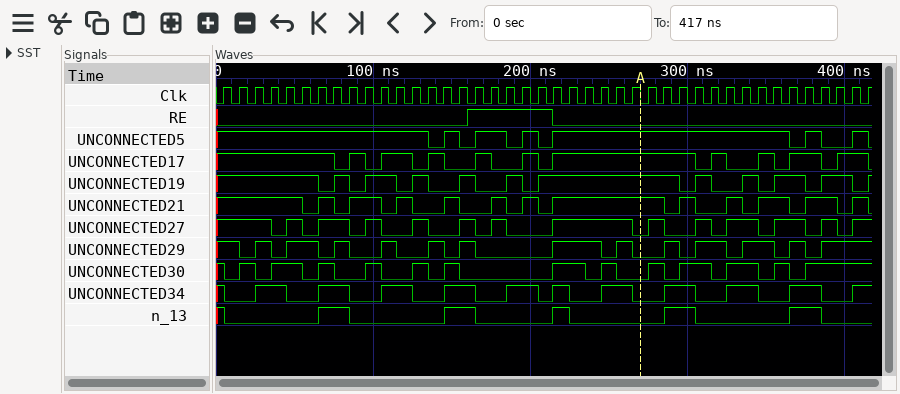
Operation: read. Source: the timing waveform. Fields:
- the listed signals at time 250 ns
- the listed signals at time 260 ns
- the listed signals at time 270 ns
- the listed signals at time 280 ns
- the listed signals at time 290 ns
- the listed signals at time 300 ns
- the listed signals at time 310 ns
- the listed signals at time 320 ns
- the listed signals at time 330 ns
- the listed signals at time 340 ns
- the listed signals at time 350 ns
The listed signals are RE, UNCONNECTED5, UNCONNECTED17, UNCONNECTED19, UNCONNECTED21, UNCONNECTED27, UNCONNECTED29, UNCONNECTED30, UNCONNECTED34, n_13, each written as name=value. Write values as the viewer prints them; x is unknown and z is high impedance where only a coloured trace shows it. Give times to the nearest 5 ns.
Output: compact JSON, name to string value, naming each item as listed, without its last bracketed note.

{"the listed signals at time 250 ns": "RE=0, UNCONNECTED5=1, UNCONNECTED17=1, UNCONNECTED19=1, UNCONNECTED21=1, UNCONNECTED27=1, UNCONNECTED29=0, UNCONNECTED30=1, UNCONNECTED34=1, n_13=0", "the listed signals at time 260 ns": "RE=0, UNCONNECTED5=1, UNCONNECTED17=1, UNCONNECTED19=1, UNCONNECTED21=1, UNCONNECTED27=1, UNCONNECTED29=1, UNCONNECTED30=0, UNCONNECTED34=1, n_13=0", "the listed signals at time 270 ns": "RE=0, UNCONNECTED5=1, UNCONNECTED17=1, UNCONNECTED19=1, UNCONNECTED21=1, UNCONNECTED27=0, UNCONNECTED29=0, UNCONNECTED30=0, UNCONNECTED34=0, n_13=0", "the listed signals at time 280 ns": "RE=0, UNCONNECTED5=1, UNCONNECTED17=1, UNCONNECTED19=1, UNCONNECTED21=1, UNCONNECTED27=1, UNCONNECTED29=0, UNCONNECTED30=1, UNCONNECTED34=0, n_13=0", "the listed signals at time 290 ns": "RE=0, UNCONNECTED5=1, UNCONNECTED17=1, UNCONNECTED19=1, UNCONNECTED21=0, UNCONNECTED27=0, UNCONNECTED29=1, UNCONNECTED30=0, UNCONNECTED34=1, n_13=1", "the listed signals at time 300 ns": "RE=0, UNCONNECTED5=1, UNCONNECTED17=1, UNCONNECTED19=0, UNCONNECTED21=1, UNCONNECTED27=0, UNCONNECTED29=0, UNCONNECTED30=1, UNCONNECTED34=1, n_13=1", "the listed signals at time 310 ns": "RE=0, UNCONNECTED5=1, UNCONNECTED17=0, UNCONNECTED19=1, UNCONNECTED21=0, UNCONNECTED27=1, UNCONNECTED29=1, UNCONNECTED30=1, UNCONNECTED34=0, n_13=0", "the listed signals at time 320 ns": "RE=0, UNCONNECTED5=1, UNCONNECTED17=1, UNCONNECTED19=0, UNCONNECTED21=0, UNCONNECTED27=0, UNCONNECTED29=1, UNCONNECTED30=0, UNCONNECTED34=0, n_13=0", "the listed signals at time 330 ns": "RE=0, UNCONNECTED5=1, UNCONNECTED17=0, UNCONNECTED19=0, UNCONNECTED21=1, UNCONNECTED27=1, UNCONNECTED29=0, UNCONNECTED30=1, UNCONNECTED34=1, n_13=0", "the listed signals at time 340 ns": "RE=0, UNCONNECTED5=1, UNCONNECTED17=0, UNCONNECTED19=1, UNCONNECTED21=0, UNCONNECTED27=1, UNCONNECTED29=1, UNCONNECTED30=1, UNCONNECTED34=1, n_13=0", "the listed signals at time 350 ns": "RE=0, UNCONNECTED5=1, UNCONNECTED17=1, UNCONNECTED19=0, UNCONNECTED21=1, UNCONNECTED27=0, UNCONNECTED29=1, UNCONNECTED30=0, UNCONNECTED34=0, n_13=0"}
